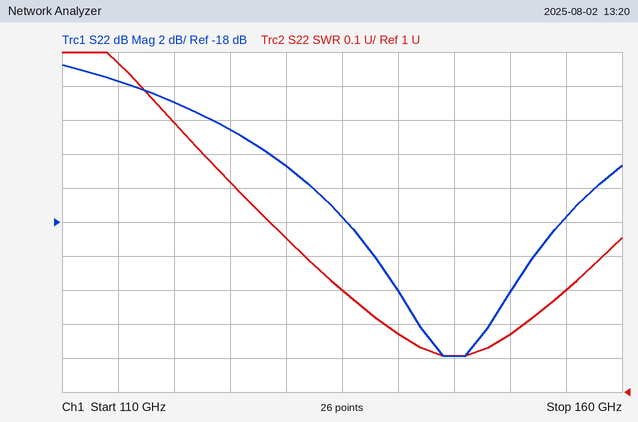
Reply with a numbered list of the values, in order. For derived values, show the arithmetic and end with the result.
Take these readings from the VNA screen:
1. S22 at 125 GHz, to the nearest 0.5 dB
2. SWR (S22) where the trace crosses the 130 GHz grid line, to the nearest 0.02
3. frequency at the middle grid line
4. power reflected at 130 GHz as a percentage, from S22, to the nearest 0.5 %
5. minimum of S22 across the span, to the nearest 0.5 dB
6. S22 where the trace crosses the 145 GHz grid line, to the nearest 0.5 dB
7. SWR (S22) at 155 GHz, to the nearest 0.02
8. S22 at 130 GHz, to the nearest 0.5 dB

1. -12.5 dB
2. 1.46
3. 135 GHz
4. 10^(-14.5/10) ≈ 3.5 %
5. -26.0 dB
6. -26.0 dB
7. 1.30
8. -14.5 dB
